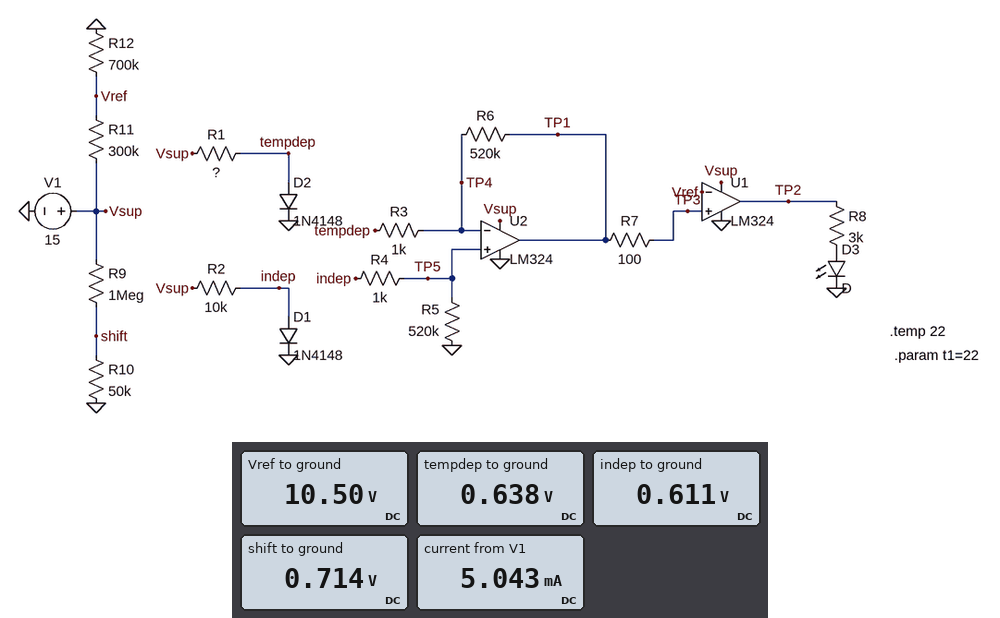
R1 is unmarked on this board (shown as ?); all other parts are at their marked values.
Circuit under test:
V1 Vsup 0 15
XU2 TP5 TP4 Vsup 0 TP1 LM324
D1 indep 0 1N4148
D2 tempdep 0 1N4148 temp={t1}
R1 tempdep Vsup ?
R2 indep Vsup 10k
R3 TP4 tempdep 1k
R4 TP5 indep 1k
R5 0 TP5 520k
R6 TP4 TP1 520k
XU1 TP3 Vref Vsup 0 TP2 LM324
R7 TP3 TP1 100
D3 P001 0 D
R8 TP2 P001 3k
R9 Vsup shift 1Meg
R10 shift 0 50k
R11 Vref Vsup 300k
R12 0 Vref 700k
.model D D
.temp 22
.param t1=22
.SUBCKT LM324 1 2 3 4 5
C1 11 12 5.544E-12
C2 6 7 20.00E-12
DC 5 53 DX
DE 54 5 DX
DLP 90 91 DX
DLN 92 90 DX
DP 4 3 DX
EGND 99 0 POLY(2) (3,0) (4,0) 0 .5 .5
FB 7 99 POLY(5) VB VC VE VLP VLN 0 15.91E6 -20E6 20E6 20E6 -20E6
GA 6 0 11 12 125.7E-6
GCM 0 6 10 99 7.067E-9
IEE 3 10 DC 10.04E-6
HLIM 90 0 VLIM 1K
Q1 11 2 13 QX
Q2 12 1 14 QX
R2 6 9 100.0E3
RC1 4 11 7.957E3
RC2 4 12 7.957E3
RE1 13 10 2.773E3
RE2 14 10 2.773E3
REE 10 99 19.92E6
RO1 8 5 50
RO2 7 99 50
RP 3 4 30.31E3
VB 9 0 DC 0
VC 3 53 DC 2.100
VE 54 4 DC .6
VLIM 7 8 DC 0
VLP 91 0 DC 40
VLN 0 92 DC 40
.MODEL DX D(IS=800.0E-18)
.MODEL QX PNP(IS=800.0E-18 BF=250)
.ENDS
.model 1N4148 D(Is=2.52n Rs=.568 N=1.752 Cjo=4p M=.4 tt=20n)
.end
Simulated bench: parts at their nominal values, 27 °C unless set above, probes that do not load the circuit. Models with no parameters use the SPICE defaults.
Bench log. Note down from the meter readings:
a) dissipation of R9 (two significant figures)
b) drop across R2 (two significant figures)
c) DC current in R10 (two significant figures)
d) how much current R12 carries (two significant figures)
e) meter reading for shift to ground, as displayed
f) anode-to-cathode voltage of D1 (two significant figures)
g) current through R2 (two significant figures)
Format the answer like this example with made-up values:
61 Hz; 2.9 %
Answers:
200 µW; 14 V; 14 µA; 15 µA; 0.714 V; 610 mV; 1.4 mA
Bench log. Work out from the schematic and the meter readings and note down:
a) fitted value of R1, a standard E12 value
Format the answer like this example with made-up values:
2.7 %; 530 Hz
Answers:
5.6 kΩ
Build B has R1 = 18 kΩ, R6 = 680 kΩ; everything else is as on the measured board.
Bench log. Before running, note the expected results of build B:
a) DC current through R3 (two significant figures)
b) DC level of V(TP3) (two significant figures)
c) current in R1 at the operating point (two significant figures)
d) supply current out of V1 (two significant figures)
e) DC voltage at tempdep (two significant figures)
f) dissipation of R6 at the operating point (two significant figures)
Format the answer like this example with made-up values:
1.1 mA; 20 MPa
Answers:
19 µA; 13 V; 800 µA; 3.3 mA; 590 mV; 240 µW
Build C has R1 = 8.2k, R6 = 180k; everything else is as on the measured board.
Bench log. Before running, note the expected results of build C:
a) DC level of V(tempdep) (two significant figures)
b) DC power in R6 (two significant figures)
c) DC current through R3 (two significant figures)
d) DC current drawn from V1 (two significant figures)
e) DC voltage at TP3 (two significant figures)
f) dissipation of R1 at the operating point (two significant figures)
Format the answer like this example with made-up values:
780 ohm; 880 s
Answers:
620 mV; 1.7 µW; 3.1 µA; 4.2 mA; 57 mV; 25 mW
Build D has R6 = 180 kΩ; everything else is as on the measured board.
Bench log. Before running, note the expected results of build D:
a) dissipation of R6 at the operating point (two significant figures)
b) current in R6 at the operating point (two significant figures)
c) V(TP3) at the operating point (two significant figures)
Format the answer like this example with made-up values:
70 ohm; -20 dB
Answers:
2.1 µW; 3.4 µA; 25 mV
